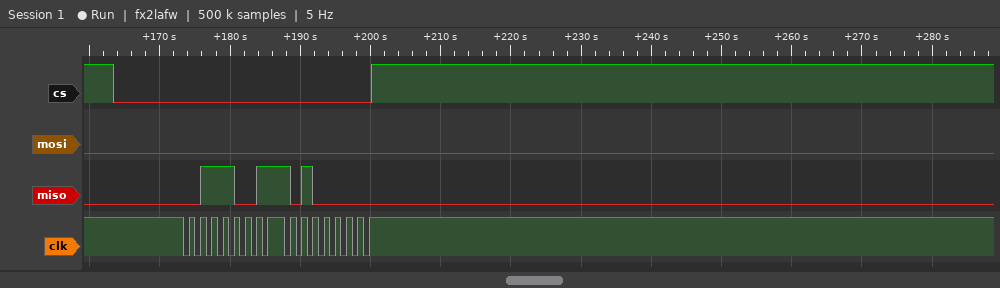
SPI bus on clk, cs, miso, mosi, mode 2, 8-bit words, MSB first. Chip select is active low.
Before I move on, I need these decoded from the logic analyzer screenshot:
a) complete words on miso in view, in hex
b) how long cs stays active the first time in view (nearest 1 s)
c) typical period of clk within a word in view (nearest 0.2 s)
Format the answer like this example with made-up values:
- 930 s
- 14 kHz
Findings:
- 39, A0
- 37 s
- 1.6 s
